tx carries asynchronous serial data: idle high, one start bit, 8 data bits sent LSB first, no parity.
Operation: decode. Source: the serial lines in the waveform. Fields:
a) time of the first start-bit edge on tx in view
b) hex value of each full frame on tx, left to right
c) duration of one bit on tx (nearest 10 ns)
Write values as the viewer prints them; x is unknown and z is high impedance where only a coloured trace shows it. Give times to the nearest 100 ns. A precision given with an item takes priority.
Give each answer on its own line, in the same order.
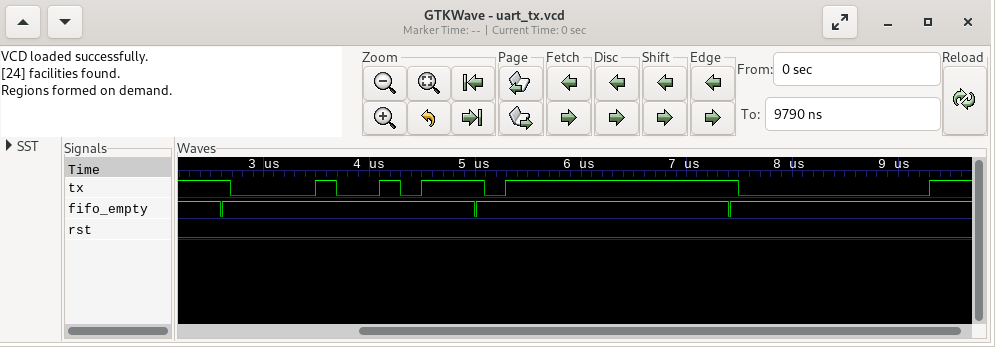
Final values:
2700 ns
48, FF, 00
200 ns
